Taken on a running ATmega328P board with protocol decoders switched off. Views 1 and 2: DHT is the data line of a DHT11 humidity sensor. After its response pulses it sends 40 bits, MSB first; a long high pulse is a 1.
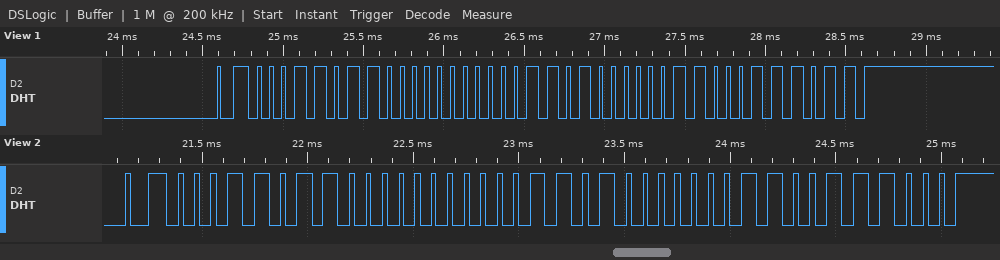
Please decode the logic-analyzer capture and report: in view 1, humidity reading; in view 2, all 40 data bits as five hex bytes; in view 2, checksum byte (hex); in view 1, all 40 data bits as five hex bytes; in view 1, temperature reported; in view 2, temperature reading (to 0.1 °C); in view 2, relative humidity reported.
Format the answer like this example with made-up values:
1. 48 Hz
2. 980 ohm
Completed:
1. 27 %
2. 1B 00 1A 03 38
3. 0x38
4. 1B 00 1A 06 3B
5. 26.6 °C
6. 26.3 °C
7. 27 %
